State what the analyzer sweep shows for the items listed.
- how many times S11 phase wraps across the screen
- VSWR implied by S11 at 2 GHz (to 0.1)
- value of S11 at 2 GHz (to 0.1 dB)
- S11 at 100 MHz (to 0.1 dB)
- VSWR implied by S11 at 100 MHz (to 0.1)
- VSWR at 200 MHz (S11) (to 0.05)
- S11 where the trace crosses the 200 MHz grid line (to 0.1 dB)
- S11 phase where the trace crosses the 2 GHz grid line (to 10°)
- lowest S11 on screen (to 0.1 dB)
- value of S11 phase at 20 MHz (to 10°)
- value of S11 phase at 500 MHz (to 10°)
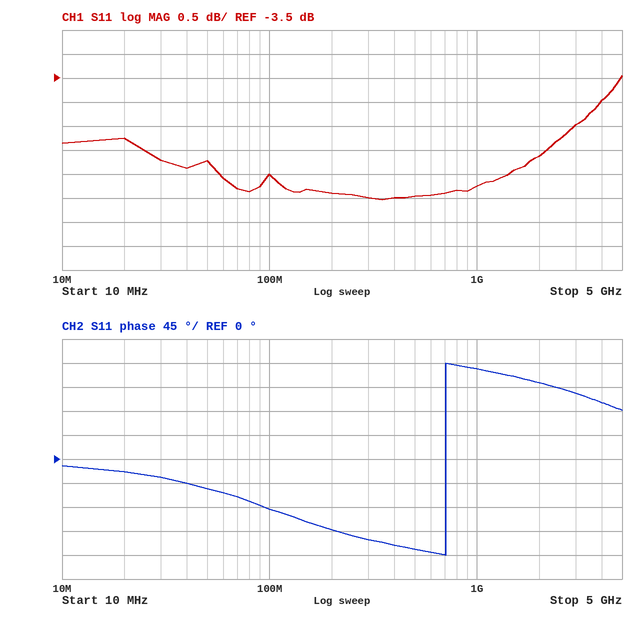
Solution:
1
3.5
-5.1 dB
-5.5 dB
3.3
3.05
-5.9 dB
140°
-6.0 dB
-20°
-170°
